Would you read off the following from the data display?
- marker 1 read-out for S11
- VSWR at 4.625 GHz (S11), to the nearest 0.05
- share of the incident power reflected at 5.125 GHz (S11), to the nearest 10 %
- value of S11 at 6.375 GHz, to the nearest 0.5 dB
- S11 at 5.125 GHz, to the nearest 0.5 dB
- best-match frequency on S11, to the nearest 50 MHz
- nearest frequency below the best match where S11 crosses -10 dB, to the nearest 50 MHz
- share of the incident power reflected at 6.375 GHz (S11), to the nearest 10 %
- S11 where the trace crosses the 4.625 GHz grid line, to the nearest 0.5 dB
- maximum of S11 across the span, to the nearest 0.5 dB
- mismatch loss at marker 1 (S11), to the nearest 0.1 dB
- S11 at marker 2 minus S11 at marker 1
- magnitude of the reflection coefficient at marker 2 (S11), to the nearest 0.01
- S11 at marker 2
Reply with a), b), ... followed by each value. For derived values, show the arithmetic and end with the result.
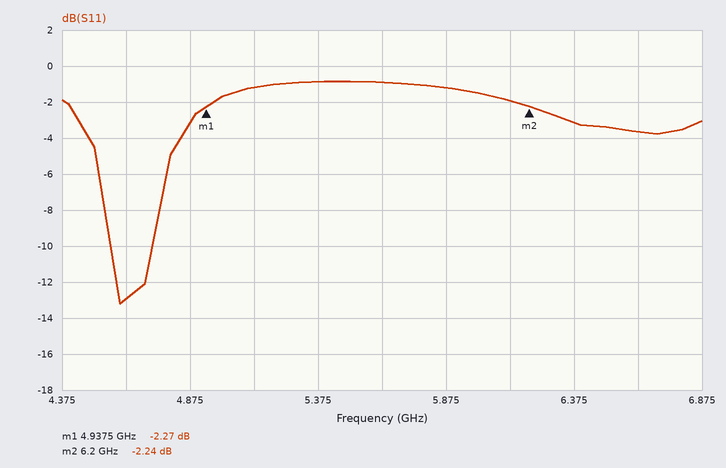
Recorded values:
a) -2.27 dB
b) |Γ| = 10^(-13/20) = 0.2239; VSWR = (1 + 0.2239)/(1 − 0.2239) ≈ 1.58, so 1.60 to the nearest 0.05
c) 10^(-1/10) ≈ 79.4 %, so 80 % to the nearest 10 %
d) -3.0 dB
e) -1.0 dB
f) 4.60 GHz
g) 4.55 GHz
h) 10^(-3/10) ≈ 50 %
i) -13.0 dB
j) -1.0 dB
k) −10 log10(1 − 10^(-2.27/10)) ≈ 3.9 dB
l) -2.24 − (-2.27) = 0.03 dB
m) 10^(-2.24/20) ≈ 0.77
n) -2.24 dB
